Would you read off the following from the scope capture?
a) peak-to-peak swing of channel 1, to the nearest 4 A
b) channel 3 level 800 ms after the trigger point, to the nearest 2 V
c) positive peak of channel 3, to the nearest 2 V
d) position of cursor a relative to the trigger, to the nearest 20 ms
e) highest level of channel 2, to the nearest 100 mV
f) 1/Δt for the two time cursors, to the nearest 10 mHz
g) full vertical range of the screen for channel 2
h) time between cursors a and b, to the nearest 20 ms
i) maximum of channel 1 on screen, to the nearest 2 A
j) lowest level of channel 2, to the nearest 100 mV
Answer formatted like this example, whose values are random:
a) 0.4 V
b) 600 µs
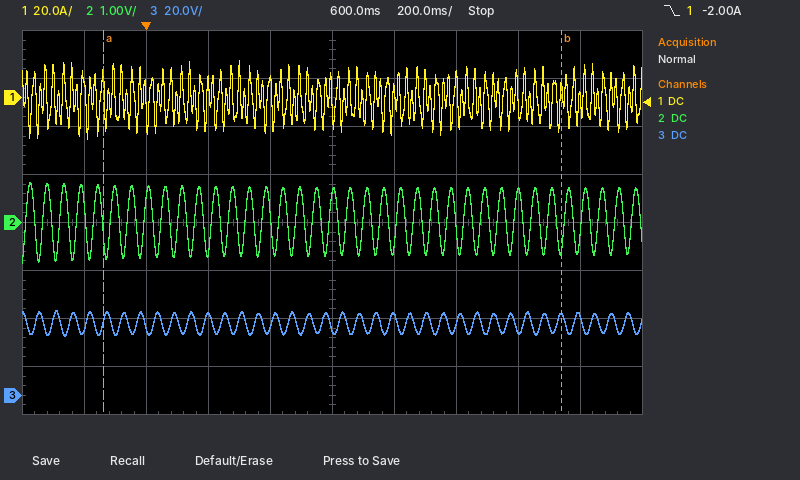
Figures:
a) 32 A
b) 32 V
c) 36 V
d) -140 ms
e) 800 mV
f) 680 mHz
g) 8 V
h) 1.48 s
i) 16 A
j) -800 mV
